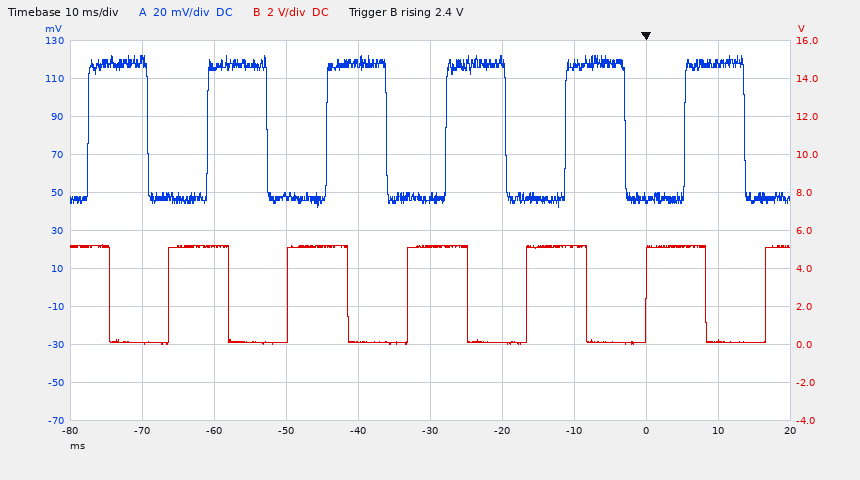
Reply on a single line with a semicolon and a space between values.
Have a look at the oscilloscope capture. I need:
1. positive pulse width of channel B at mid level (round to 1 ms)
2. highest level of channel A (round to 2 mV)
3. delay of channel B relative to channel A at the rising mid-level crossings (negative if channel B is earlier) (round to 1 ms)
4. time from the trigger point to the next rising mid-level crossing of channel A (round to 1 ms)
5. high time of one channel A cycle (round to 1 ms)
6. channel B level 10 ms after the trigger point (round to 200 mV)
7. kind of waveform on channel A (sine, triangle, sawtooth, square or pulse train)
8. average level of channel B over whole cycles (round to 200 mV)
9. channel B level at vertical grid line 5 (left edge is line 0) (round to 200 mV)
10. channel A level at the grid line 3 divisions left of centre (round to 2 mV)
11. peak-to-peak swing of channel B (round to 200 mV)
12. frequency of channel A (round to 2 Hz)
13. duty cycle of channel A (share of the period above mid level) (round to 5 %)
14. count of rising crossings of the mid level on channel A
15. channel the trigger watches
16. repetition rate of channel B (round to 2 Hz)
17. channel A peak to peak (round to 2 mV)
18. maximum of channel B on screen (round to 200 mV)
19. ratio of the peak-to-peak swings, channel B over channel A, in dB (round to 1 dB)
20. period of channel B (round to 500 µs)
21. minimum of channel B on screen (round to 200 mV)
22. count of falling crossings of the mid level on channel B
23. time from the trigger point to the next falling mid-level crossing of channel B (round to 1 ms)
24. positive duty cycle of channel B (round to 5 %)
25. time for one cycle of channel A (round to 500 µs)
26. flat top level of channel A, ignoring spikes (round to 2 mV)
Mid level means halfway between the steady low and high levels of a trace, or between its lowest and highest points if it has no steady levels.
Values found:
8 ms; 122 mV; -5 ms; 5 ms; 8 ms; 200 mV; square; 2.6 V; 5.2 V; 116 mV; 5.2 V; 60 Hz; 50 %; 6; channel B; 60 Hz; 80 mV; 5.2 V; 36 dB; 16.5 ms; 0.0 V; 6; 8 ms; 50 %; 16.5 ms; 118 mV
